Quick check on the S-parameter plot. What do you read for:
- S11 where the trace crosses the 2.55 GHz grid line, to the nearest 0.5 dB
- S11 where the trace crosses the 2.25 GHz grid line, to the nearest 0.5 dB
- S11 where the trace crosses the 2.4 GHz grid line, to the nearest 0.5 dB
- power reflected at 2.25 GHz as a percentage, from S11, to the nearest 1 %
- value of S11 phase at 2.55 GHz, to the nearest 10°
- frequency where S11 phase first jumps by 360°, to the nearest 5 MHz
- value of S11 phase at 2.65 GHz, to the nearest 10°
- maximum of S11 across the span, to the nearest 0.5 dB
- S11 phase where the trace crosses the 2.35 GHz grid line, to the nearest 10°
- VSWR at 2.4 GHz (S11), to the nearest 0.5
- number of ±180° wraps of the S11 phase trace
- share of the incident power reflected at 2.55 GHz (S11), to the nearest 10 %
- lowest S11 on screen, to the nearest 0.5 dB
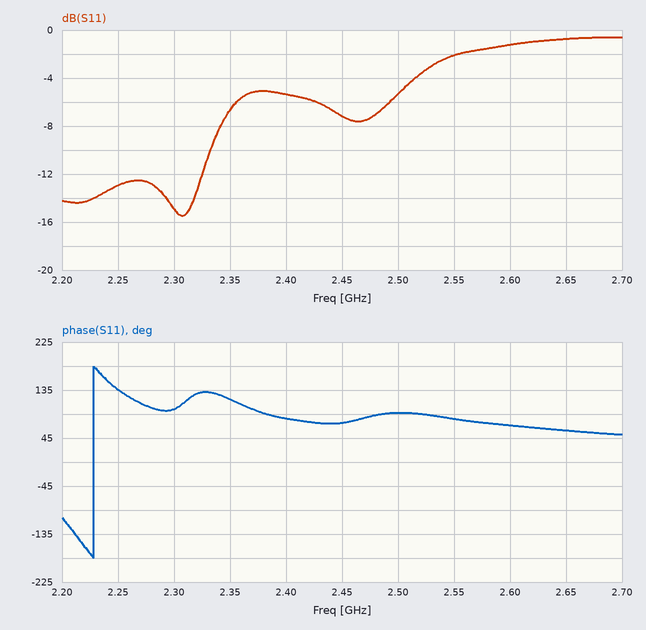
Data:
-2.0 dB
-13.0 dB
-5.5 dB
5 %
80°
2.230 GHz
60°
-0.5 dB
120°
3.5
1
60 %
-15.5 dB
